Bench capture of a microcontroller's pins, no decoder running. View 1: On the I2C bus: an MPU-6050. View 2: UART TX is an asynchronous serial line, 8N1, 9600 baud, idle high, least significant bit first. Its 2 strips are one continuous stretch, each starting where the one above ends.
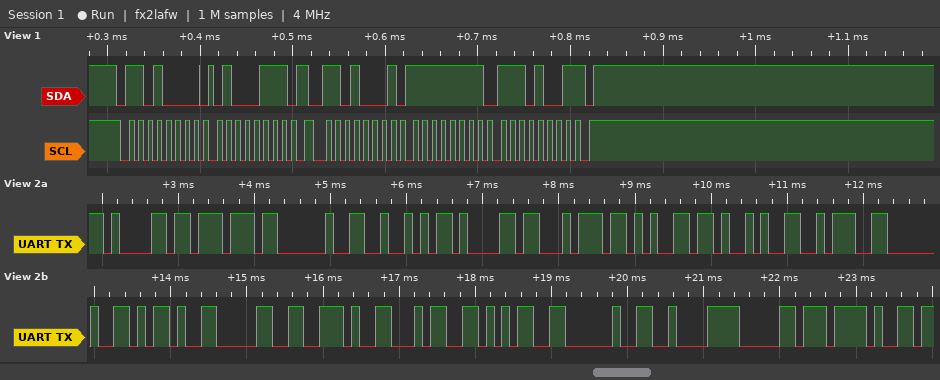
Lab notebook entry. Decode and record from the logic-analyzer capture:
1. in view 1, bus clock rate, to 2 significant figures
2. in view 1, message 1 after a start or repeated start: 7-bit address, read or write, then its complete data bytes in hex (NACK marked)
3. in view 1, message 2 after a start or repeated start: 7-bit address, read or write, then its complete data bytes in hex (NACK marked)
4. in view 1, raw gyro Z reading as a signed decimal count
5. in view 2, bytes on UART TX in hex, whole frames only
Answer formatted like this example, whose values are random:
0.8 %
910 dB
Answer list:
100 kHz
0x68 write: 47
0x68 read: FF E9 NACK
-23
61 77 20 52 61 74 65 29 3A 20 2D 30 2E 34 35 20 C2 B0 2F
